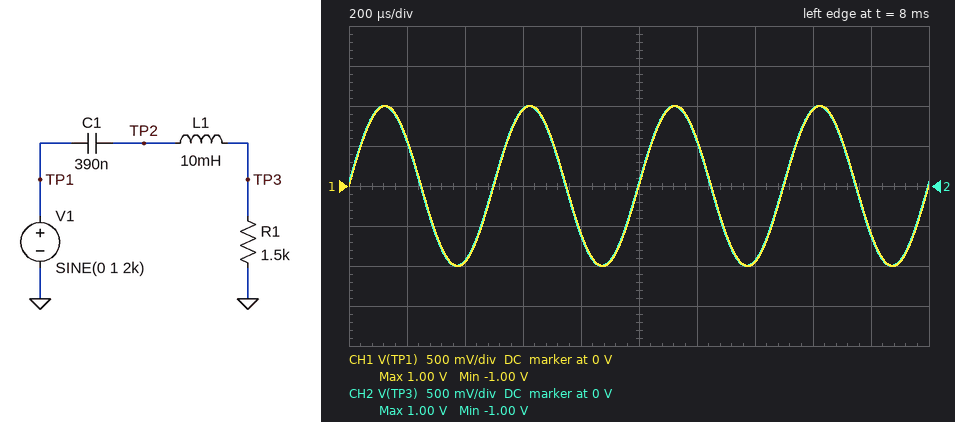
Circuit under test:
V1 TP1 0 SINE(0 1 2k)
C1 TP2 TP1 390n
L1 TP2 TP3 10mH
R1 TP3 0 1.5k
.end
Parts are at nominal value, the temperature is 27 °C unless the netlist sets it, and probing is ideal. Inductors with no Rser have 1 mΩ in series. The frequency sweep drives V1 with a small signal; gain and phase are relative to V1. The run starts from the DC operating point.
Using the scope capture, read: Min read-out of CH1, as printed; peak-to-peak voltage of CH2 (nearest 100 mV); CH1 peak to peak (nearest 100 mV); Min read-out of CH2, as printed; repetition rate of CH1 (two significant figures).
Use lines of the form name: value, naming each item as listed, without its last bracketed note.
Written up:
Min read-out of CH1, as printed: -1.00 V
peak-to-peak voltage of CH2: 2.0 V
CH1 peak to peak: 2.0 V
Min read-out of CH2, as printed: -1.00 V
repetition rate of CH1: 2.0 kHz
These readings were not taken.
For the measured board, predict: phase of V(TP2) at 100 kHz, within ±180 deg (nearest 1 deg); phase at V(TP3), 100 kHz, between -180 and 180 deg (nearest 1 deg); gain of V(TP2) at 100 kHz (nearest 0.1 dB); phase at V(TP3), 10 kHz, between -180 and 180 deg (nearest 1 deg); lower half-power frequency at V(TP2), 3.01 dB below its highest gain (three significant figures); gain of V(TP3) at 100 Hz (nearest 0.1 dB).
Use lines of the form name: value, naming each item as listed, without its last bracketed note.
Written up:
phase of V(TP2) at 100 kHz, within ±180 deg: 0 deg
phase at V(TP3), 100 kHz, between -180 and 180 deg: -77 deg
gain of V(TP2) at 100 kHz: 0 dB
phase at V(TP3), 10 kHz, between -180 and 180 deg: -21 deg
lower half-power frequency at V(TP2), 3.01 dB below its highest gain: 274 Hz
gain of V(TP3) at 100 Hz: -9.2 dB
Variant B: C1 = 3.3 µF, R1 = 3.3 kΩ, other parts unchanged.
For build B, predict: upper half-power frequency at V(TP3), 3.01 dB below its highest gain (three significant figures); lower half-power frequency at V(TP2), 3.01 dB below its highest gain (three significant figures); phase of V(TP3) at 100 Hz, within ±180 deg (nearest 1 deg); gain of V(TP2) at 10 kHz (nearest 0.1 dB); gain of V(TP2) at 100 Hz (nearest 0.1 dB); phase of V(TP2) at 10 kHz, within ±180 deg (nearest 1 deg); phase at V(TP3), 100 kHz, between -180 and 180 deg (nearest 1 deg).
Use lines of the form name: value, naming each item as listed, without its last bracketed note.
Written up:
upper half-power frequency at V(TP3), 3.01 dB below its highest gain: 52.5 kHz
lower half-power frequency at V(TP2), 3.01 dB below its highest gain: 14.6 Hz
phase of V(TP3) at 100 Hz, within ±180 deg: 8 deg
gain of V(TP2) at 10 kHz: 0 dB
gain of V(TP2) at 100 Hz: -0.1 dB
phase of V(TP2) at 10 kHz, within ±180 deg: 0 deg
phase at V(TP3), 100 kHz, between -180 and 180 deg: -62 deg
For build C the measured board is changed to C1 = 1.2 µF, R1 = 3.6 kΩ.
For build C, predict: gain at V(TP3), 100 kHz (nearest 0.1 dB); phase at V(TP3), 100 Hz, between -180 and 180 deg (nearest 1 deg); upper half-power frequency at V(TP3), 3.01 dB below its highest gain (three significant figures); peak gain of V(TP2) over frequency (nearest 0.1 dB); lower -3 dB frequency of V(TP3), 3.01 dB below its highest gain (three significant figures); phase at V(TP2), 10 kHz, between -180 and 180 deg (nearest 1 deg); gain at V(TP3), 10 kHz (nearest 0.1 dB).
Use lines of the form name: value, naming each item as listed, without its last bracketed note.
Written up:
gain at V(TP3), 100 kHz: -6.1 dB
phase at V(TP3), 100 Hz, between -180 and 180 deg: 20 deg
upper half-power frequency at V(TP3), 3.01 dB below its highest gain: 57.3 kHz
peak gain of V(TP2) over frequency: 0 dB
lower -3 dB frequency of V(TP3), 3.01 dB below its highest gain: 36.8 Hz
phase at V(TP2), 10 kHz, between -180 and 180 deg: 0 deg
gain at V(TP3), 10 kHz: -0.1 dB
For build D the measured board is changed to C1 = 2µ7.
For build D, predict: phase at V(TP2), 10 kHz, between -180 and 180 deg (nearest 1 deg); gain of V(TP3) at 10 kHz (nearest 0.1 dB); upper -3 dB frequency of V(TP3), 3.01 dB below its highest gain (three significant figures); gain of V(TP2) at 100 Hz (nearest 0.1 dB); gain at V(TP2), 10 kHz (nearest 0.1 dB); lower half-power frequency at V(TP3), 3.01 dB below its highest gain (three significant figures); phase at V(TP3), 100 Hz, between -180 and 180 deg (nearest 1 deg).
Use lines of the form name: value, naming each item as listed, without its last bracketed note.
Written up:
phase at V(TP2), 10 kHz, between -180 and 180 deg: 0 deg
gain of V(TP3) at 10 kHz: -0.7 dB
upper -3 dB frequency of V(TP3), 3.01 dB below its highest gain: 23.9 kHz
gain of V(TP2) at 100 Hz: -0.6 dB
gain at V(TP2), 10 kHz: 0 dB
lower half-power frequency at V(TP3), 3.01 dB below its highest gain: 39.2 Hz
phase at V(TP3), 100 Hz, between -180 and 180 deg: 21 deg
